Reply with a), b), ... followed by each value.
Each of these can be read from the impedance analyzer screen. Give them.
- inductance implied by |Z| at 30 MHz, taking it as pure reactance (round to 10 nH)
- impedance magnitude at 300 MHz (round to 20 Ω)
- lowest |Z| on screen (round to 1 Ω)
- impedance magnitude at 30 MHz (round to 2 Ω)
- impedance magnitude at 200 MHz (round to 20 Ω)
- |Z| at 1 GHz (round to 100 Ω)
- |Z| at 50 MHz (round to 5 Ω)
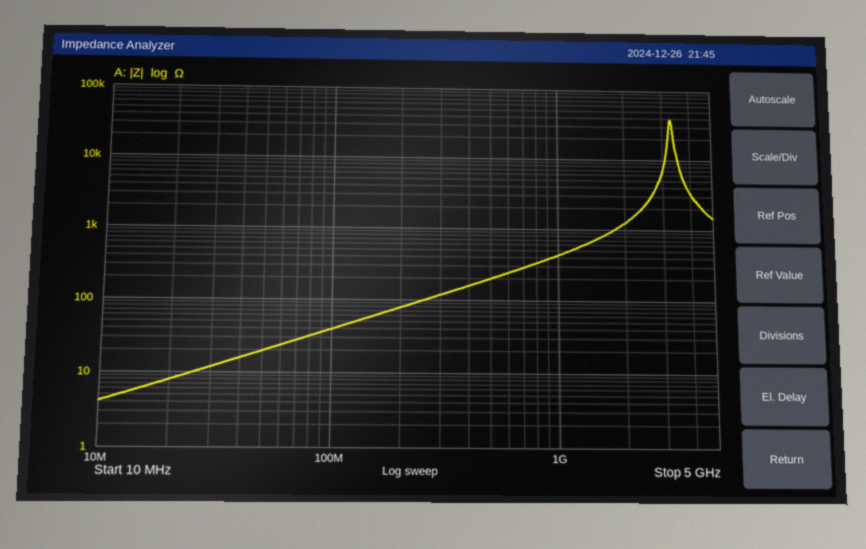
a) 60 nH
b) 120 Ω
c) 4 Ω
d) 12 Ω
e) 80 Ω
f) 400 Ω
g) 20 Ω
